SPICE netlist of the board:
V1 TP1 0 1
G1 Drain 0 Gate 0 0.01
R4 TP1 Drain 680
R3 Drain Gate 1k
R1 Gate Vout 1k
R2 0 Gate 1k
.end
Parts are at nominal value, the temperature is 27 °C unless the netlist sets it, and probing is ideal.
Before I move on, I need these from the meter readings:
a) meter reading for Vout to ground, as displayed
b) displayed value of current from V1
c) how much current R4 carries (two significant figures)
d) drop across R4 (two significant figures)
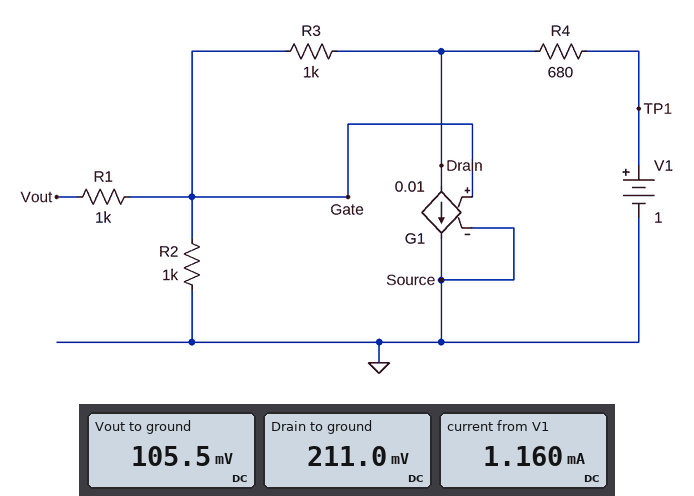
105.5 mV
1.160 mA
1.2 mA
790 mV
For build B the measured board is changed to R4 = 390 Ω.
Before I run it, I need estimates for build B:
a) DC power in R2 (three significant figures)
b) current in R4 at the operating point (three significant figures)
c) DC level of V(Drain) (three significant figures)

25.3 µW
1.75 mA
318 mV
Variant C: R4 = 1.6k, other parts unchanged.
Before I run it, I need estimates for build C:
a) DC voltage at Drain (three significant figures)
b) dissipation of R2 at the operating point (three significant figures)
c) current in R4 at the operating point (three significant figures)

102 mV
2.60 µW
561 µA
